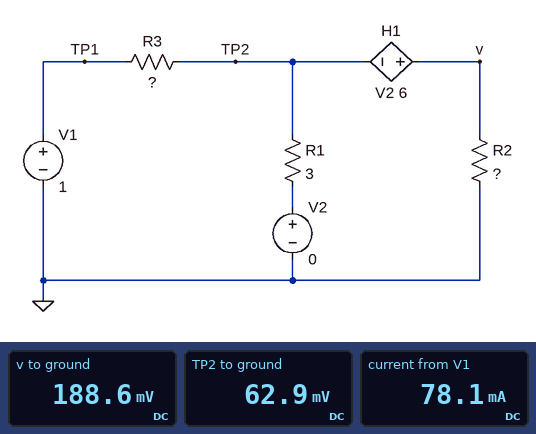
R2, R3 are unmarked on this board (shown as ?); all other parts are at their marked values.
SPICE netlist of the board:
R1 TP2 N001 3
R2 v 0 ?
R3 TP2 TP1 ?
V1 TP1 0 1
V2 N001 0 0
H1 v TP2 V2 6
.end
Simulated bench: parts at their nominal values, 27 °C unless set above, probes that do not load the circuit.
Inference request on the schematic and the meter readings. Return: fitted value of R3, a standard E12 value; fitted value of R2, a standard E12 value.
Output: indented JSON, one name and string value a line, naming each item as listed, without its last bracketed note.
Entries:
{
  "fitted value of R3, a standard E12 value": "12 Ω",
  "fitted value of R2, a standard E12 value": "3.3 Ω"
}
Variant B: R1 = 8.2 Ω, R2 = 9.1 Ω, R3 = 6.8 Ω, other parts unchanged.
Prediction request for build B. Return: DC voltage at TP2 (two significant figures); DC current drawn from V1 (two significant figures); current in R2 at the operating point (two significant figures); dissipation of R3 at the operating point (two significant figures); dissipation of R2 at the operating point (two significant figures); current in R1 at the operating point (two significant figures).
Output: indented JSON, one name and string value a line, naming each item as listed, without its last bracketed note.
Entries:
{
  "DC voltage at TP2": "320 mV",
  "DC current drawn from V1": "100 mA",
  "current in R2 at the operating point": "61 mA",
  "dissipation of R3 at the operating point": "68 mW",
  "dissipation of R2 at the operating point": "34 mW",
  "current in R1 at the operating point": "39 mA"
}
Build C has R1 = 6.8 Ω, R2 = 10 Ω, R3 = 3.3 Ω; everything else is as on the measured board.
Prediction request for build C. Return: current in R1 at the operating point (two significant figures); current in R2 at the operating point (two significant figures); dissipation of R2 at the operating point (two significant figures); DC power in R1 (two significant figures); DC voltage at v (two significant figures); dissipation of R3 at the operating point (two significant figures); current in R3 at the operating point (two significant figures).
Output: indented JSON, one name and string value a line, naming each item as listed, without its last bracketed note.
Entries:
{
  "current in R1 at the operating point": "70 mA",
  "current in R2 at the operating point": "89 mA",
  "dissipation of R2 at the operating point": "80 mW",
  "DC power in R1": "33 mW",
  "DC voltage at v": "890 mV",
  "dissipation of R3 at the operating point": "84 mW",
  "current in R3 at the operating point": "160 mA"
}
